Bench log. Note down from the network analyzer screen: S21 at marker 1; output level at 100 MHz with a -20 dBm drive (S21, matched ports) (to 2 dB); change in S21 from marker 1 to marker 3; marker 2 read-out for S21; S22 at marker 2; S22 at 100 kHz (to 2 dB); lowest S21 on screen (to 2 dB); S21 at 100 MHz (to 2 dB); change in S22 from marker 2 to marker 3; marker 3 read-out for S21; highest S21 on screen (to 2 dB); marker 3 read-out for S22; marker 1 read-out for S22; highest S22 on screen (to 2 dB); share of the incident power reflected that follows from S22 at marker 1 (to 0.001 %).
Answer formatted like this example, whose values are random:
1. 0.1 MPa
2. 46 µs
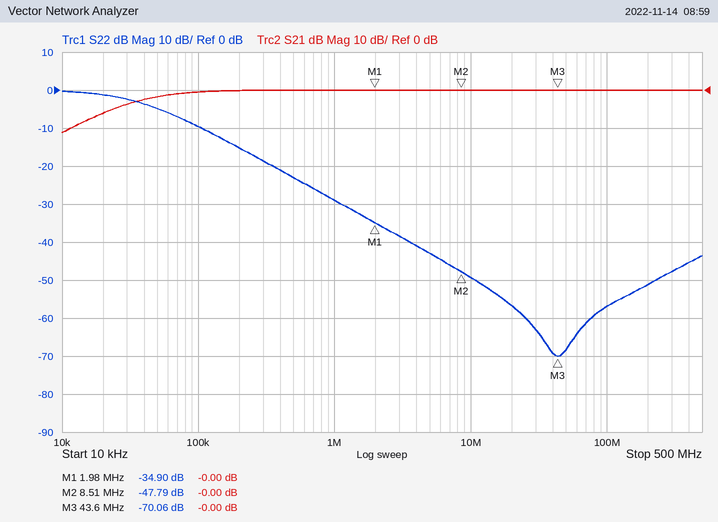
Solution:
1. -0.00 dB
2. -20 dBm
3. 0.00 dB
4. -0.00 dB
5. -47.79 dB
6. -10 dB
7. -12 dB
8. 0 dB
9. -22.27 dB
10. -0.00 dB
11. 0 dB
12. -70.06 dB
13. -34.90 dB
14. 0 dB
15. 0.032 %
